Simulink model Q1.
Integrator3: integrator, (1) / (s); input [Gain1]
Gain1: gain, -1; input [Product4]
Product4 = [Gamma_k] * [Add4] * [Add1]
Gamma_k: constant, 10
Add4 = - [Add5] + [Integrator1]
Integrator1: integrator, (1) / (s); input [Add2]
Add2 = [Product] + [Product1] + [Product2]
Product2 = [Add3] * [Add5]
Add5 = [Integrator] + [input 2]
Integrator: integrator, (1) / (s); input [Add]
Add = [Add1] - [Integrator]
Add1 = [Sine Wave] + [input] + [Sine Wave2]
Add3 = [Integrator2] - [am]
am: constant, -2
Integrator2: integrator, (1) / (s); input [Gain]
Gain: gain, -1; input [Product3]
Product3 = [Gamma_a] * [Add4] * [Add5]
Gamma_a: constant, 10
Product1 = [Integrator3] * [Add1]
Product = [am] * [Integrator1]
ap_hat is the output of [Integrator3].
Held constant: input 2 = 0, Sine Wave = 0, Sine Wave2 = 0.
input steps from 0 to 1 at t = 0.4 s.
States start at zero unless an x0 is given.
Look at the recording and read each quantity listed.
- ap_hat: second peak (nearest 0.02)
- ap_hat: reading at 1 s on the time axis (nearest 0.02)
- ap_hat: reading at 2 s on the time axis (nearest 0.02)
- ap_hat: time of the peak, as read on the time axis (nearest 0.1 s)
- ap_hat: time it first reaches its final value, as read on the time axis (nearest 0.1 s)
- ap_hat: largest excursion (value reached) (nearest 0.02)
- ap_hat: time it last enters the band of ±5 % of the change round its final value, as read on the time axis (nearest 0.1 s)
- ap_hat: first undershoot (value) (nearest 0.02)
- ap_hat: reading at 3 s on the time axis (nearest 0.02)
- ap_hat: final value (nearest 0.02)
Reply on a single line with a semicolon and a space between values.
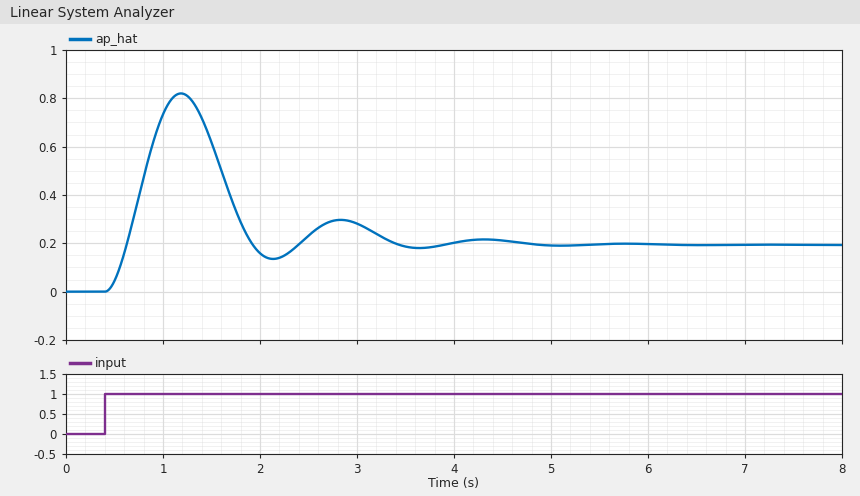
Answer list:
0.30; 0.74; 0.16; 1.2 s; 0.6 s; 0.82; 4.7 s; 0.14; 0.28; 0.20
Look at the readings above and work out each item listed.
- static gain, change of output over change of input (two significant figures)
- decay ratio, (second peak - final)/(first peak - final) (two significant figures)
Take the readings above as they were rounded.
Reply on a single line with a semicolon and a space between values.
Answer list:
0.20; 0.16
